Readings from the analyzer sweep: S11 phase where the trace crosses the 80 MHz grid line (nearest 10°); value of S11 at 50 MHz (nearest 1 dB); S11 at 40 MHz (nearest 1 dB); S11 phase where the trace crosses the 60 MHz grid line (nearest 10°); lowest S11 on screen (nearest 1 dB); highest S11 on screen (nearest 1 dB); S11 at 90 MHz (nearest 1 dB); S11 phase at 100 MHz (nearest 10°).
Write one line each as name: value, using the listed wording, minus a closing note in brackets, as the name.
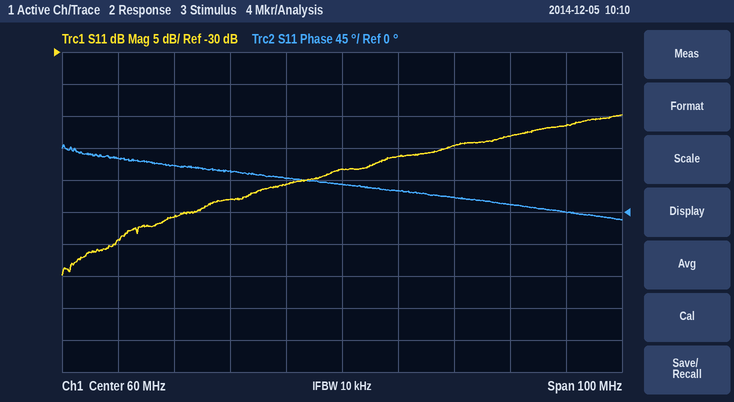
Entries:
S11 phase where the trace crosses the 80 MHz grid line: 20°
value of S11 at 50 MHz: -51 dB
S11 at 40 MHz: -53 dB
S11 phase where the trace crosses the 60 MHz grid line: 40°
lowest S11 on screen: -65 dB
highest S11 on screen: -40 dB
S11 at 90 MHz: -43 dB
S11 phase at 100 MHz: 0°
